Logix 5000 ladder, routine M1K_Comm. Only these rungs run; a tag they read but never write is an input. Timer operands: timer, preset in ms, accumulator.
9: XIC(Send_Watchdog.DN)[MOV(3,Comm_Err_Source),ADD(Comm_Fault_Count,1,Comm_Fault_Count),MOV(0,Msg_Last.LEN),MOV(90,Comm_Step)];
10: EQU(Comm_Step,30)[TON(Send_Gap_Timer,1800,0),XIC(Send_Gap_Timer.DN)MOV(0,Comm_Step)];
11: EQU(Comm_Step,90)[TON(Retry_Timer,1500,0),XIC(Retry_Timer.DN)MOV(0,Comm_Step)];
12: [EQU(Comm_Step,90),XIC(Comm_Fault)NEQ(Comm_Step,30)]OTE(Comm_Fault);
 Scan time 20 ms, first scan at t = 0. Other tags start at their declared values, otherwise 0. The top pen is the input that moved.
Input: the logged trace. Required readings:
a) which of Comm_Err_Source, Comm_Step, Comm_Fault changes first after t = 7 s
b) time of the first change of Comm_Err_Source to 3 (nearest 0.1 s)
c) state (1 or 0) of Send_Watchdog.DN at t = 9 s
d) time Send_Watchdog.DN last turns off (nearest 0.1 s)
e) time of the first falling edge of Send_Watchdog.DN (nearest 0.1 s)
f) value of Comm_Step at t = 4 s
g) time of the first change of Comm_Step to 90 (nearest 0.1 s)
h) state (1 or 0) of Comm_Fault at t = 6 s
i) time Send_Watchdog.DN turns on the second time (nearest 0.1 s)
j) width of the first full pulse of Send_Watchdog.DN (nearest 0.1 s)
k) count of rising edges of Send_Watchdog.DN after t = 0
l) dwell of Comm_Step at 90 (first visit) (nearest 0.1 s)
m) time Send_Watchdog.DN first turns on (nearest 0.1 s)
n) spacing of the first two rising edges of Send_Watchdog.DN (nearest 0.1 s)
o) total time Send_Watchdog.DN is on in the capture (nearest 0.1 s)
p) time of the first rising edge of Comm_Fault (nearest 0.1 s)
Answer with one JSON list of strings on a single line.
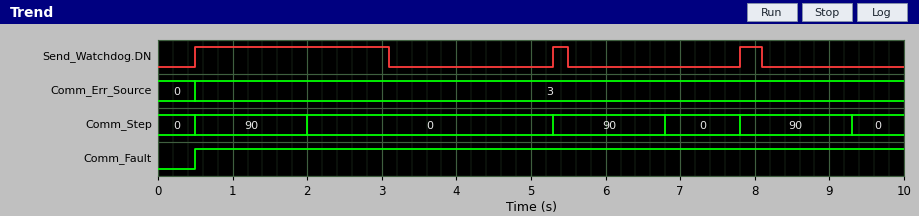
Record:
["Comm_Step", "0.5 s", "0", "8.1 s", "3.1 s", "0", "0.5 s", "1", "5.3 s", "2.6 s", "3", "1.5 s", "0.5 s", "4.8 s", "3.1 s", "0.5 s"]
